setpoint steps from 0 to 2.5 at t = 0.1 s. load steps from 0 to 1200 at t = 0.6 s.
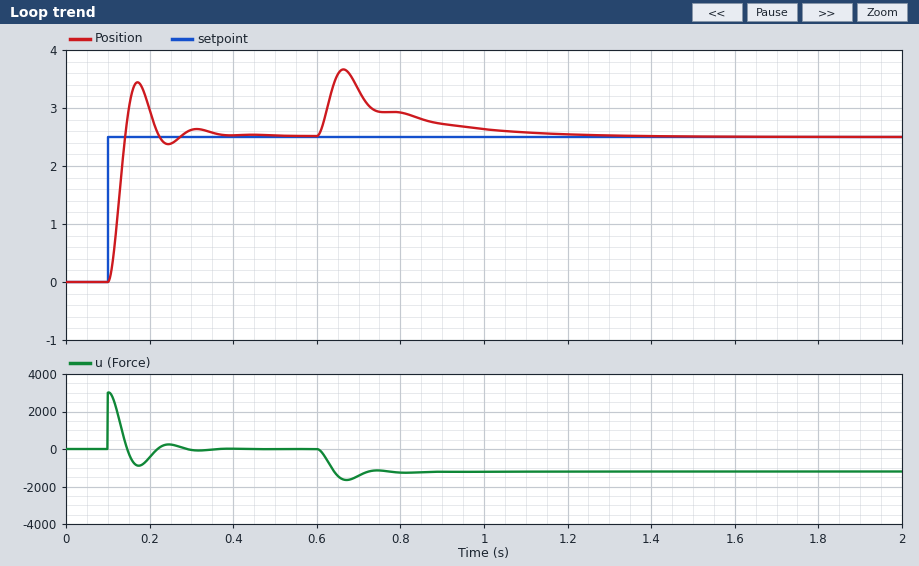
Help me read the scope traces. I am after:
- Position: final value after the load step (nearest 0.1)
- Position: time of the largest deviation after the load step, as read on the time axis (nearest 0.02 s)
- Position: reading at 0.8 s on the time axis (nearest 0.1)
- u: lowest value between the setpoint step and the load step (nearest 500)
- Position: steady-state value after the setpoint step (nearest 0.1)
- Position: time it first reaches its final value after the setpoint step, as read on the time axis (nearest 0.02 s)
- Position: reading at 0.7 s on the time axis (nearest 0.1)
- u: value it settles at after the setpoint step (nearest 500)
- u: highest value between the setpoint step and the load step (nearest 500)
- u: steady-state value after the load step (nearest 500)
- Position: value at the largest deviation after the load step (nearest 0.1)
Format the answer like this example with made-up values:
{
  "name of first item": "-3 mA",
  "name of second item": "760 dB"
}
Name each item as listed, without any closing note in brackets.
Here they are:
{
  "Position: final value after the load step": "2.5",
  "Position: time of the largest deviation after the load step, as read on the time axis": "0.66 s",
  "Position: reading at 0.8 s on the time axis": "2.9",
  "u: lowest value between the setpoint step and the load step": "-1000",
  "Position: steady-state value after the setpoint step": "2.5",
  "Position: time it first reaches its final value after the setpoint step, as read on the time axis": "0.14 s",
  "Position: reading at 0.7 s on the time axis": "3.3",
  "u: value it settles at after the setpoint step": "0",
  "u: highest value between the setpoint step and the load step": "3000",
  "u: steady-state value after the load step": "-1000",
  "Position: value at the largest deviation after the load step": "3.7"
}
